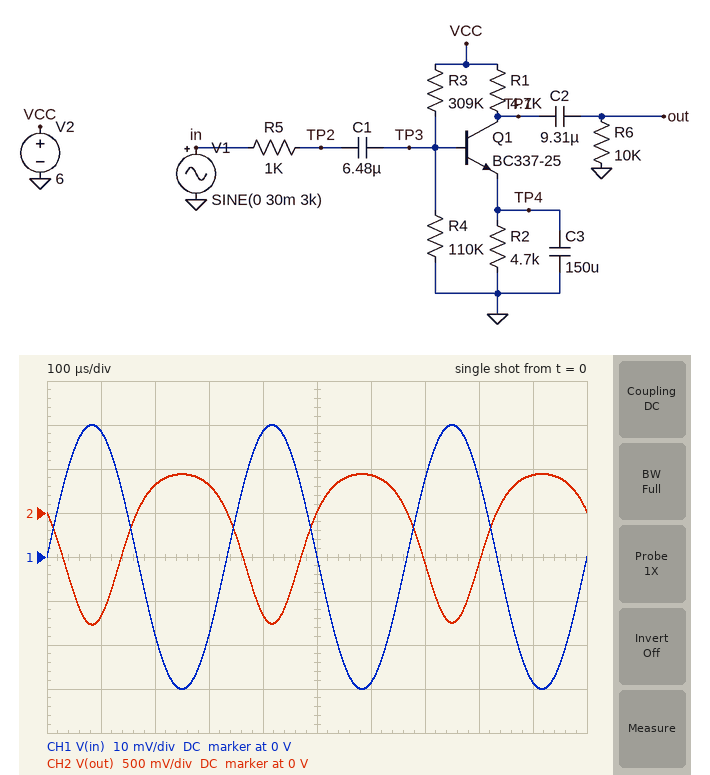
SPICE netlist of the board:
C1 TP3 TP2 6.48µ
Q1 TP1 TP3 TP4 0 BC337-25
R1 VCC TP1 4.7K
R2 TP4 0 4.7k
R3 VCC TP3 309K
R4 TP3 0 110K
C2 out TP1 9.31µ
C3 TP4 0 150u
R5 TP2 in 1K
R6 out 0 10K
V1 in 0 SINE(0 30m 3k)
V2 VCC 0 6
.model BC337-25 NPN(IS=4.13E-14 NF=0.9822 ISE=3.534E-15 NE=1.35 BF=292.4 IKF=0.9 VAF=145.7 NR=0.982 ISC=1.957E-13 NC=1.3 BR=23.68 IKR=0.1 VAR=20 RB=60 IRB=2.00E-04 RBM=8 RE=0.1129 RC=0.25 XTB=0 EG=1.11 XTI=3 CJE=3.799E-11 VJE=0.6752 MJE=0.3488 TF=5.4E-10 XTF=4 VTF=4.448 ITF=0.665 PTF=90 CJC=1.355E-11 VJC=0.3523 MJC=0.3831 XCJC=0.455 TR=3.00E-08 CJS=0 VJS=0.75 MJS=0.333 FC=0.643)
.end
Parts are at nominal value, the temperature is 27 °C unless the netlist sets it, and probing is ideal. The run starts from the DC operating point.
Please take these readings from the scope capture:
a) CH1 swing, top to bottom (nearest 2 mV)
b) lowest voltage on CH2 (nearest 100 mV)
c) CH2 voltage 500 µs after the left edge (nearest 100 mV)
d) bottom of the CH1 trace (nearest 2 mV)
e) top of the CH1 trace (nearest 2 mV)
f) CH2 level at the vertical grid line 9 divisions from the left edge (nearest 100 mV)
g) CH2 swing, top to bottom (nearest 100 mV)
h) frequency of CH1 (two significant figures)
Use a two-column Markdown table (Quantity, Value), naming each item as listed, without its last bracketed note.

| Quantity | Value |
|---|---|
| CH1 swing, top to bottom | 60 mV |
| lowest voltage on CH2 | -1.3 V |
| CH2 voltage 500 µs after the left edge | 0 V |
| bottom of the CH1 trace | -30 mV |
| top of the CH1 trace | 30 mV |
| CH2 level at the vertical grid line 9 divisions from the left edge | 400 mV |
| CH2 swing, top to bottom | 1.7 V |
| frequency of CH1 | 3.0 kHz |
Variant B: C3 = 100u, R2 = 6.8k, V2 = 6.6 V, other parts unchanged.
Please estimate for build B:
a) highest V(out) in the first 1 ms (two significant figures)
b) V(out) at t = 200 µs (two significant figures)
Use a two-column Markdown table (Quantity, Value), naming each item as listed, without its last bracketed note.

| Quantity | Value |
|---|---|
| highest V(out) in the first 1 ms | 360 mV |
| V(out) at t = 200 µs | 260 mV |
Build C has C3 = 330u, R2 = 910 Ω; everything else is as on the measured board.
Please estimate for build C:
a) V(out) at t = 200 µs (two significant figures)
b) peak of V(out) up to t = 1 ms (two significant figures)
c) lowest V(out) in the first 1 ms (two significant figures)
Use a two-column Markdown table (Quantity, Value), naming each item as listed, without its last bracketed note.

| Quantity | Value |
|---|---|
| V(out) at t = 200 µs | 1.2 V |
| peak of V(out) up to t = 1 ms | 1.7 V |
| lowest V(out) in the first 1 ms | -1.4 V |
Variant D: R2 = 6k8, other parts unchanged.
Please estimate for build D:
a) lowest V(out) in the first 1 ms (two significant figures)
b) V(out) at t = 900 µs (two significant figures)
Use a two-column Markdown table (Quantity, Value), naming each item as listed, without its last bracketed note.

| Quantity | Value |
|---|---|
| lowest V(out) in the first 1 ms | -930 mV |
| V(out) at t = 900 µs | 310 mV |
